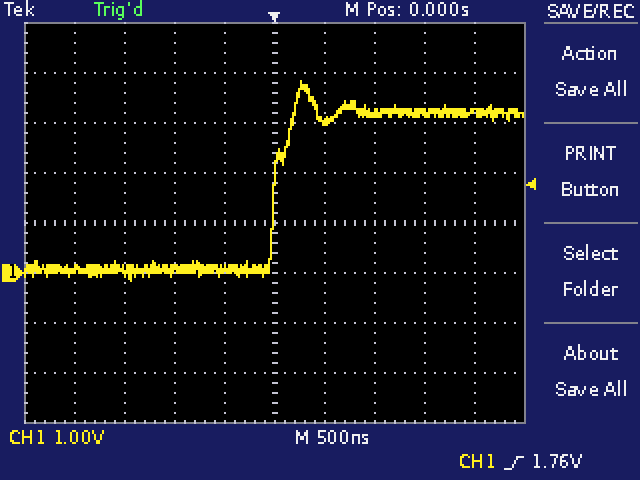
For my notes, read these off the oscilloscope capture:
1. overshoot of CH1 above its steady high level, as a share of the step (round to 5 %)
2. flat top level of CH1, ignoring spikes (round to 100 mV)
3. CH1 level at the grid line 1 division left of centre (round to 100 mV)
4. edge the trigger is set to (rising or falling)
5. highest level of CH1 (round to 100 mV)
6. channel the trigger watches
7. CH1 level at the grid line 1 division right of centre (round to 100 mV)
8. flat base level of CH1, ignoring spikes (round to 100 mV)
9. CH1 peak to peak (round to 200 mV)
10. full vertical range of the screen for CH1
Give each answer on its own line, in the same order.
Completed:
20 %
3.2 V
100 mV
rising
3.8 V
CH1
3.0 V
100 mV
4.0 V
8 V
